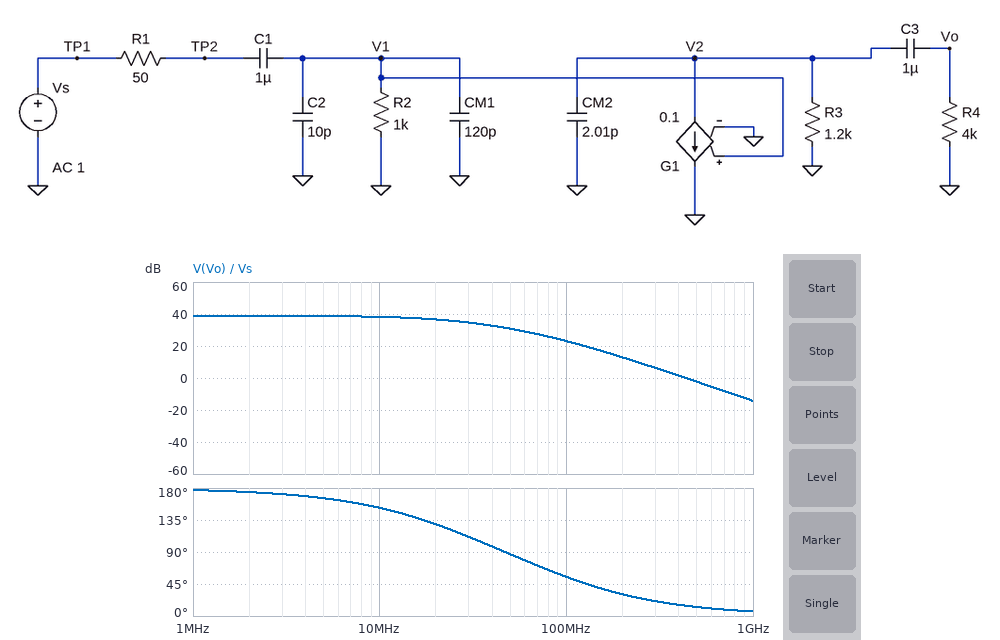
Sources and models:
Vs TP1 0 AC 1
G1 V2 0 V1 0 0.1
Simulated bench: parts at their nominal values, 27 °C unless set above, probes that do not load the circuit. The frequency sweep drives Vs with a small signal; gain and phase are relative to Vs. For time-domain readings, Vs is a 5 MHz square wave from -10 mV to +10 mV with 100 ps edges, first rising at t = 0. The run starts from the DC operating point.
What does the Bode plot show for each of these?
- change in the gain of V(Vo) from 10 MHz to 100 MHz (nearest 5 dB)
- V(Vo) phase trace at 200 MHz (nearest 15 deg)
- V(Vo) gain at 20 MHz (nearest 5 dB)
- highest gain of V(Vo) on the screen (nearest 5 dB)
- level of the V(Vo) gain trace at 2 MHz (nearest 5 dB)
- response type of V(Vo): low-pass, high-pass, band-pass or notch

-15 dB
30 deg
35 dB
40 dB
40 dB
low-pass
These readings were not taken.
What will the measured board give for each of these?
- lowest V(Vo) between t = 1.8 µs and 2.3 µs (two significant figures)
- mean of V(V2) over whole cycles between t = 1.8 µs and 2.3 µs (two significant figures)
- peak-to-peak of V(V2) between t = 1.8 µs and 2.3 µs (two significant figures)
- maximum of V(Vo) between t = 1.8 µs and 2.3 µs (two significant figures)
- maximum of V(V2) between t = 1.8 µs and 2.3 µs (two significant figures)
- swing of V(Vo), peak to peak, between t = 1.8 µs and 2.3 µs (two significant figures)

-1.8 V
-880 mV
1.8 V
2.2 mV
1.7 mV
1.8 V
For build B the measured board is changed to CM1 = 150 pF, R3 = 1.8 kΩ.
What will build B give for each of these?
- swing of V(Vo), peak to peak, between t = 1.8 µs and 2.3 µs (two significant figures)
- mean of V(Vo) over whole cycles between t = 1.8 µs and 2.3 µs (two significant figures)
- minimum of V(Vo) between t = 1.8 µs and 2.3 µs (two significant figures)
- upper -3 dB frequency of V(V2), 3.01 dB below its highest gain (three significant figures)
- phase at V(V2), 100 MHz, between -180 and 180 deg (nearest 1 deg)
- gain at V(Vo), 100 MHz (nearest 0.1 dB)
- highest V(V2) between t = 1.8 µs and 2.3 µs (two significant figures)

2.4 V
-1.2 V
-2.4 V
19.1 MHz
44 deg
22.3 dB
2.3 mV
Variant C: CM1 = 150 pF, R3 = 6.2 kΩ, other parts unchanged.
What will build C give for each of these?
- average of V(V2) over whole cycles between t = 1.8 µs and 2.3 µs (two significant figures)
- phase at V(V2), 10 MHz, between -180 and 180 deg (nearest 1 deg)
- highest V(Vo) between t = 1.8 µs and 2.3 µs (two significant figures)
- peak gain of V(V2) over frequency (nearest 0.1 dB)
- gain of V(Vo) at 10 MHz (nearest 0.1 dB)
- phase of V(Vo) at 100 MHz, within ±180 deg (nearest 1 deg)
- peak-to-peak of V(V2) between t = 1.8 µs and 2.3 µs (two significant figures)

-2.3 V
137 deg
5.3 mV
47.3 dB
46.0 dB
30 deg
4.6 V
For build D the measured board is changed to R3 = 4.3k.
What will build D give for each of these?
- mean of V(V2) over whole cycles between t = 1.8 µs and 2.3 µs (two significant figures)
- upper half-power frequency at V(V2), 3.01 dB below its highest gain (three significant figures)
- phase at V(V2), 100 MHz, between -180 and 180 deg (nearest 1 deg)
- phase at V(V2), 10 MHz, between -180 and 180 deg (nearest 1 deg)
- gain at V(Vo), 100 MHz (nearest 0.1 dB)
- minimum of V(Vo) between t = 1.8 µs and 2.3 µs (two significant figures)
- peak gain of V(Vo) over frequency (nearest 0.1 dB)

-2.0 V
19.6 MHz
35 deg
144 deg
24.9 dB
-3.9 V
45.9 dB
